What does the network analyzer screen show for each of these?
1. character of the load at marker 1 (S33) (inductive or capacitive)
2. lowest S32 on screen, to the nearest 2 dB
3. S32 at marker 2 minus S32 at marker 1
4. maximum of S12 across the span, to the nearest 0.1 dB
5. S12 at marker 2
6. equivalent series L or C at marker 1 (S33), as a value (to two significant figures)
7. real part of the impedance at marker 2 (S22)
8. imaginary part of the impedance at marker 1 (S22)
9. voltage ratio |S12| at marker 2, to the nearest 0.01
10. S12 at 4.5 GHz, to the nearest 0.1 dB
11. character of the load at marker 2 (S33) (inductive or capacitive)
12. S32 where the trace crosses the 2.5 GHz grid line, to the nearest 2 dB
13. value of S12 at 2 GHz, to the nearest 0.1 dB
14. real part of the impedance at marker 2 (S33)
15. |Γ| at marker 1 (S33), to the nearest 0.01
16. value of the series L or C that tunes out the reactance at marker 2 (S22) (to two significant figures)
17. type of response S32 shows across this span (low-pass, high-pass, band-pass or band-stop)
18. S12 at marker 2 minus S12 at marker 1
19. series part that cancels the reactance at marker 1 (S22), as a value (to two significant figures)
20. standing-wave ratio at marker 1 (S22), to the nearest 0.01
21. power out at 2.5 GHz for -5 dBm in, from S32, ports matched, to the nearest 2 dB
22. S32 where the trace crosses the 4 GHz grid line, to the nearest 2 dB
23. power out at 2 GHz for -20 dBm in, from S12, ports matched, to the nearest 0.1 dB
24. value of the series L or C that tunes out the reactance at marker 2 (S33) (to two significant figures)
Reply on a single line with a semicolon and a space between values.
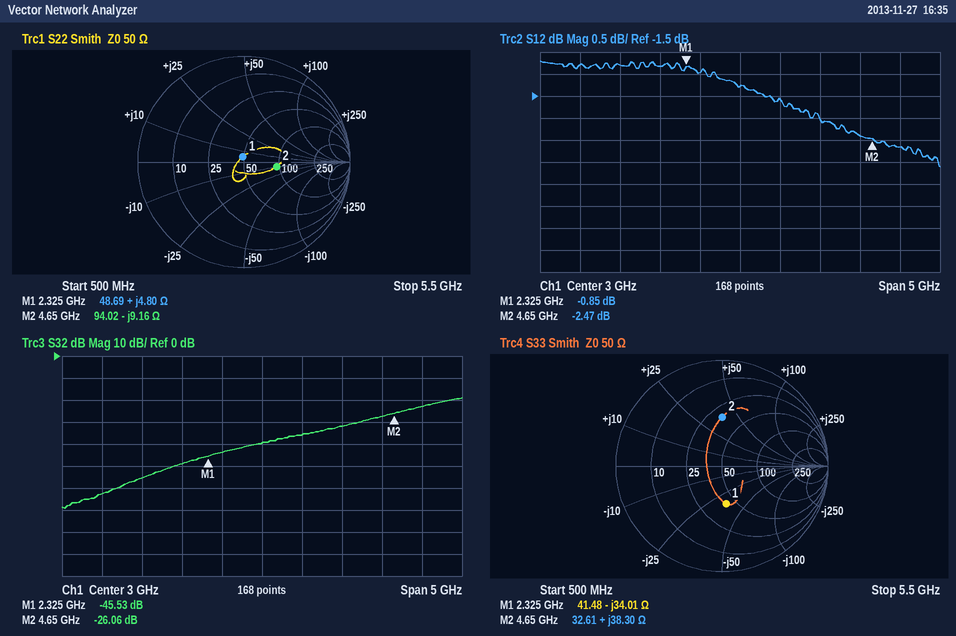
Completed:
capacitive; -70 dB; 19.47 dB; -0.7 dB; -2.47 dB; 2.0 pF; 94.02 Ω; +4.80 Ω; 0.75; -2.4 dB; inductive; -44 dB; -0.8 dB; 32.61 Ω; 0.36; 310 pH; high-pass; -1.62 dB; 14 pF; 1.11; -48 dBm; -32 dB; -20.8 dBm; 890 fF
